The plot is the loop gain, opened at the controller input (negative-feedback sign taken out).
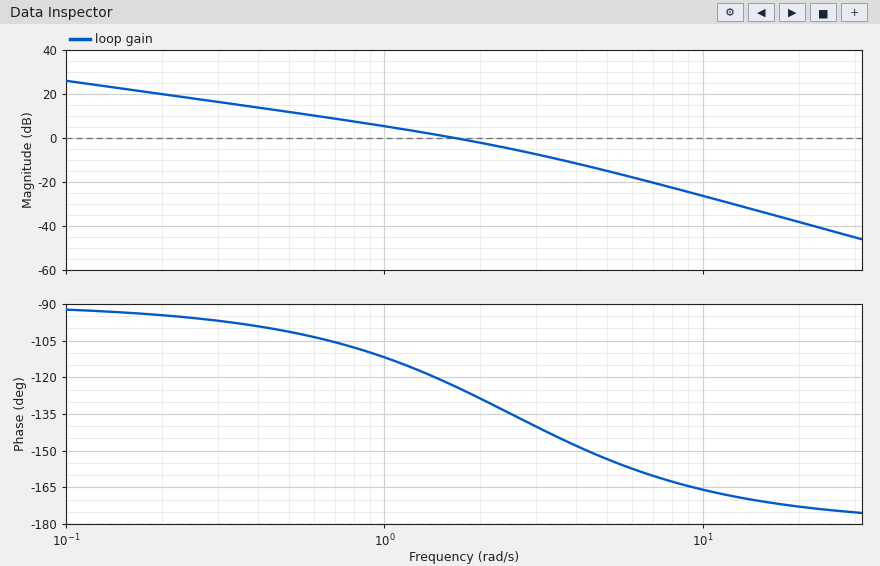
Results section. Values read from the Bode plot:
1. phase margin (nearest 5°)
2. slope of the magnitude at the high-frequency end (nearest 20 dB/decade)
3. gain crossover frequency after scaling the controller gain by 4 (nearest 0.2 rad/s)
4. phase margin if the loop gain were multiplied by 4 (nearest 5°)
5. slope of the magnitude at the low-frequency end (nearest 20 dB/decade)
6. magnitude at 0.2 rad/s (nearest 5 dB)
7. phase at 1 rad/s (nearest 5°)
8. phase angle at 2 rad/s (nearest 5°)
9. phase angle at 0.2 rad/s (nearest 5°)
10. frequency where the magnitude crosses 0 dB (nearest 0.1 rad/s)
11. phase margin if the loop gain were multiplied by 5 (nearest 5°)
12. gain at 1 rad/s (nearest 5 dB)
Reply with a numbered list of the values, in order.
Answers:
1. 55°
2. -40 dB/decade
3. 4.2 rad/s
4. 30°
5. -20 dB/decade
6. 20 dB
7. -110°
8. -130°
9. -95°
10. 1.7 rad/s
11. 30°
12. 5 dB
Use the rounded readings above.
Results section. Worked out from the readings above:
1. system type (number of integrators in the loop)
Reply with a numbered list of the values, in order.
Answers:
1. 1
